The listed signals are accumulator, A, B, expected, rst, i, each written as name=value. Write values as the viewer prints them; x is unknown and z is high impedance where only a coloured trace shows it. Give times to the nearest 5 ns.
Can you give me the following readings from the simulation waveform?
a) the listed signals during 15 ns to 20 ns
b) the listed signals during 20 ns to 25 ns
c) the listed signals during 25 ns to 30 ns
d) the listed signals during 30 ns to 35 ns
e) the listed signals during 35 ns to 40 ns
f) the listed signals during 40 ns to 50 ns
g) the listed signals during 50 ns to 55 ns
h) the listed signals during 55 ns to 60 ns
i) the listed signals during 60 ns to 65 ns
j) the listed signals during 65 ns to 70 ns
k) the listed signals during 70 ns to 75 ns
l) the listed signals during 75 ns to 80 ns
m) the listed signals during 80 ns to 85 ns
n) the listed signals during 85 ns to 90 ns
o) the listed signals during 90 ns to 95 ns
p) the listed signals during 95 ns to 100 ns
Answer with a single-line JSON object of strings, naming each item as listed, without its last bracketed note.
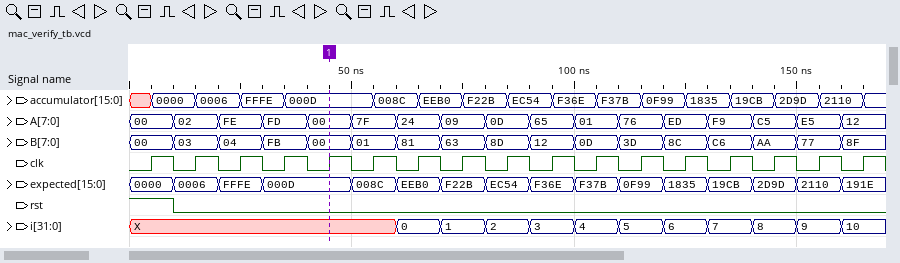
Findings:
{"the listed signals during 15 ns to 20 ns": "accumulator=0006, A=02, B=03, expected=0006, rst=0, i=X", "the listed signals during 20 ns to 25 ns": "accumulator=0006, A=FE, B=04, expected=FFFE, rst=0, i=X", "the listed signals during 25 ns to 30 ns": "accumulator=FFFE, A=FE, B=04, expected=FFFE, rst=0, i=X", "the listed signals during 30 ns to 35 ns": "accumulator=FFFE, A=FD, B=FB, expected=000D, rst=0, i=X", "the listed signals during 35 ns to 40 ns": "accumulator=000D, A=FD, B=FB, expected=000D, rst=0, i=X", "the listed signals during 40 ns to 50 ns": "accumulator=000D, A=00, B=00, expected=000D, rst=0, i=X", "the listed signals during 50 ns to 55 ns": "accumulator=000D, A=7F, B=01, expected=008C, rst=0, i=X", "the listed signals during 55 ns to 60 ns": "accumulator=008C, A=7F, B=01, expected=008C, rst=0, i=X", "the listed signals during 60 ns to 65 ns": "accumulator=008C, A=24, B=81, expected=EEB0, rst=0, i=0", "the listed signals during 65 ns to 70 ns": "accumulator=EEB0, A=24, B=81, expected=EEB0, rst=0, i=0", "the listed signals during 70 ns to 75 ns": "accumulator=EEB0, A=09, B=63, expected=F22B, rst=0, i=1", "the listed signals during 75 ns to 80 ns": "accumulator=F22B, A=09, B=63, expected=F22B, rst=0, i=1", "the listed signals during 80 ns to 85 ns": "accumulator=F22B, A=0D, B=8D, expected=EC54, rst=0, i=2", "the listed signals during 85 ns to 90 ns": "accumulator=EC54, A=0D, B=8D, expected=EC54, rst=0, i=2", "the listed signals during 90 ns to 95 ns": "accumulator=EC54, A=65, B=12, expected=F36E, rst=0, i=3", "the listed signals during 95 ns to 100 ns": "accumulator=F36E, A=65, B=12, expected=F36E, rst=0, i=3"}
